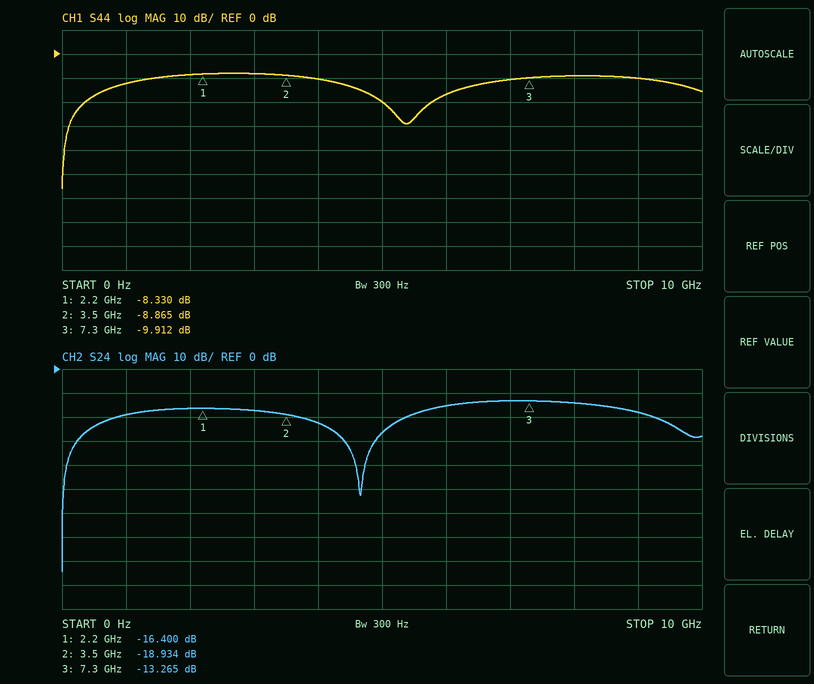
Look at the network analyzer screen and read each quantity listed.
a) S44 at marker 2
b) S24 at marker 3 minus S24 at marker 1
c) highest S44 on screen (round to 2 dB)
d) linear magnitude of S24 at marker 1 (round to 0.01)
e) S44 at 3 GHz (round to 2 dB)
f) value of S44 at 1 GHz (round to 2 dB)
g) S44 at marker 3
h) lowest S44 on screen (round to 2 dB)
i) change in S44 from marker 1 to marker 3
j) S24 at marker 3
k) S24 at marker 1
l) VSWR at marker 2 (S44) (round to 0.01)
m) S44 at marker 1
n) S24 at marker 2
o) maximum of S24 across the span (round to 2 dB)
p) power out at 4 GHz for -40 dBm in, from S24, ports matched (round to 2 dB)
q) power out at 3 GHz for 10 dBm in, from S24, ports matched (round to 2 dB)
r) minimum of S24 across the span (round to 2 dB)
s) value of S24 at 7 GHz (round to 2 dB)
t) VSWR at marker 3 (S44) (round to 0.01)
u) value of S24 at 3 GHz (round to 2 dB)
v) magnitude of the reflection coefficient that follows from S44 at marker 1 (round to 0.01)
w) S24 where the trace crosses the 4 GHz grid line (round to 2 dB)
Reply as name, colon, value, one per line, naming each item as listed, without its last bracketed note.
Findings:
S44 at marker 2: -8.865 dB
S24 at marker 3 minus S24 at marker 1: 3.135 dB
highest S44 on screen: -8 dB
linear magnitude of S24 at marker 1: 0.15
S44 at 3 GHz: -8 dB
value of S44 at 1 GHz: -12 dB
S44 at marker 3: -9.912 dB
lowest S44 on screen: -56 dB
change in S44 from marker 1 to marker 3: -1.582 dB
S24 at marker 3: -13.265 dB
S24 at marker 1: -16.400 dB
VSWR at marker 2 (S44): 2.13
S44 at marker 1: -8.330 dB
S24 at marker 2: -18.934 dB
maximum of S24 across the span: -14 dB
power out at 4 GHz for -40 dBm in, from S24, ports matched: -62 dBm
power out at 3 GHz for 10 dBm in, from S24, ports matched: -8 dBm
minimum of S24 across the span: -84 dB
value of S24 at 7 GHz: -14 dB
VSWR at marker 3 (S44): 1.94
value of S24 at 3 GHz: -18 dB
magnitude of the reflection coefficient that follows from S44 at marker 1: 0.38
S24 where the trace crosses the 4 GHz grid line: -22 dB
